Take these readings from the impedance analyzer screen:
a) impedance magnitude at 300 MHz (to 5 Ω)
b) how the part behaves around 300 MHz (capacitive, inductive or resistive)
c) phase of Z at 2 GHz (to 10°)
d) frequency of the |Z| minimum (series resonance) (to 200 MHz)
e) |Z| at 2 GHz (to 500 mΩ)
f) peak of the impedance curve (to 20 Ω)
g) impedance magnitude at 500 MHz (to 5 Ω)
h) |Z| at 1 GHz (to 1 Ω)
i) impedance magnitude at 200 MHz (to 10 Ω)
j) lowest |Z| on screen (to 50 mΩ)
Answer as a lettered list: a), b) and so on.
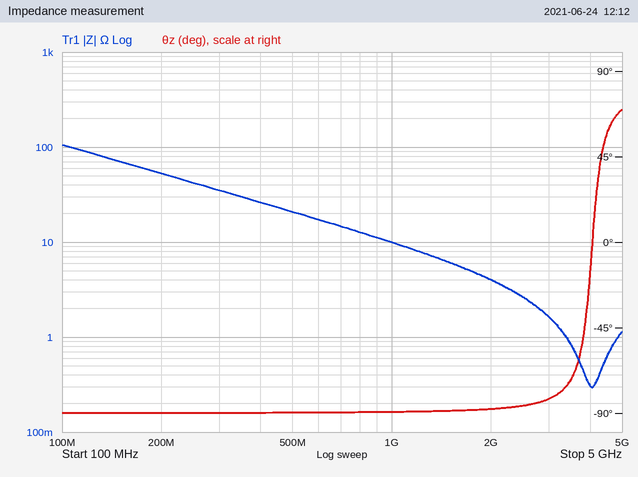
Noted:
a) 35 Ω
b) capacitive
c) -90°
d) 4.0 GHz
e) 4.0 Ω
f) 100 Ω
g) 20 Ω
h) 10 Ω
i) 50 Ω
j) 300 mΩ
